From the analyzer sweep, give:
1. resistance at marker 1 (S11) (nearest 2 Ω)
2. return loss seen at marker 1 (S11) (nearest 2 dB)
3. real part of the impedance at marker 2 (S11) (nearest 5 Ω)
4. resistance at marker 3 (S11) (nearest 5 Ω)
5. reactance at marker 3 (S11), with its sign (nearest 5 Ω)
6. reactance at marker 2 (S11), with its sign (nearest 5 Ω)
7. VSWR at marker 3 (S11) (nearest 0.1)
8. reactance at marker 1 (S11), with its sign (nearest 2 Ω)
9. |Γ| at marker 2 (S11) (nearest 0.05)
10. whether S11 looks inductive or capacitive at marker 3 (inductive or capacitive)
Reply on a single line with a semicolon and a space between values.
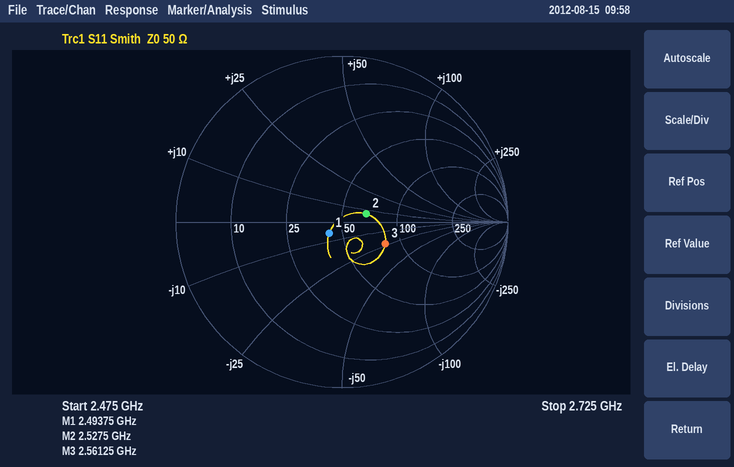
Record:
42 Ω; 20 dB; 65 Ω; 80 Ω; -25 Ω; +5 Ω; 1.8; -6 Ω; 0.15; capacitive
